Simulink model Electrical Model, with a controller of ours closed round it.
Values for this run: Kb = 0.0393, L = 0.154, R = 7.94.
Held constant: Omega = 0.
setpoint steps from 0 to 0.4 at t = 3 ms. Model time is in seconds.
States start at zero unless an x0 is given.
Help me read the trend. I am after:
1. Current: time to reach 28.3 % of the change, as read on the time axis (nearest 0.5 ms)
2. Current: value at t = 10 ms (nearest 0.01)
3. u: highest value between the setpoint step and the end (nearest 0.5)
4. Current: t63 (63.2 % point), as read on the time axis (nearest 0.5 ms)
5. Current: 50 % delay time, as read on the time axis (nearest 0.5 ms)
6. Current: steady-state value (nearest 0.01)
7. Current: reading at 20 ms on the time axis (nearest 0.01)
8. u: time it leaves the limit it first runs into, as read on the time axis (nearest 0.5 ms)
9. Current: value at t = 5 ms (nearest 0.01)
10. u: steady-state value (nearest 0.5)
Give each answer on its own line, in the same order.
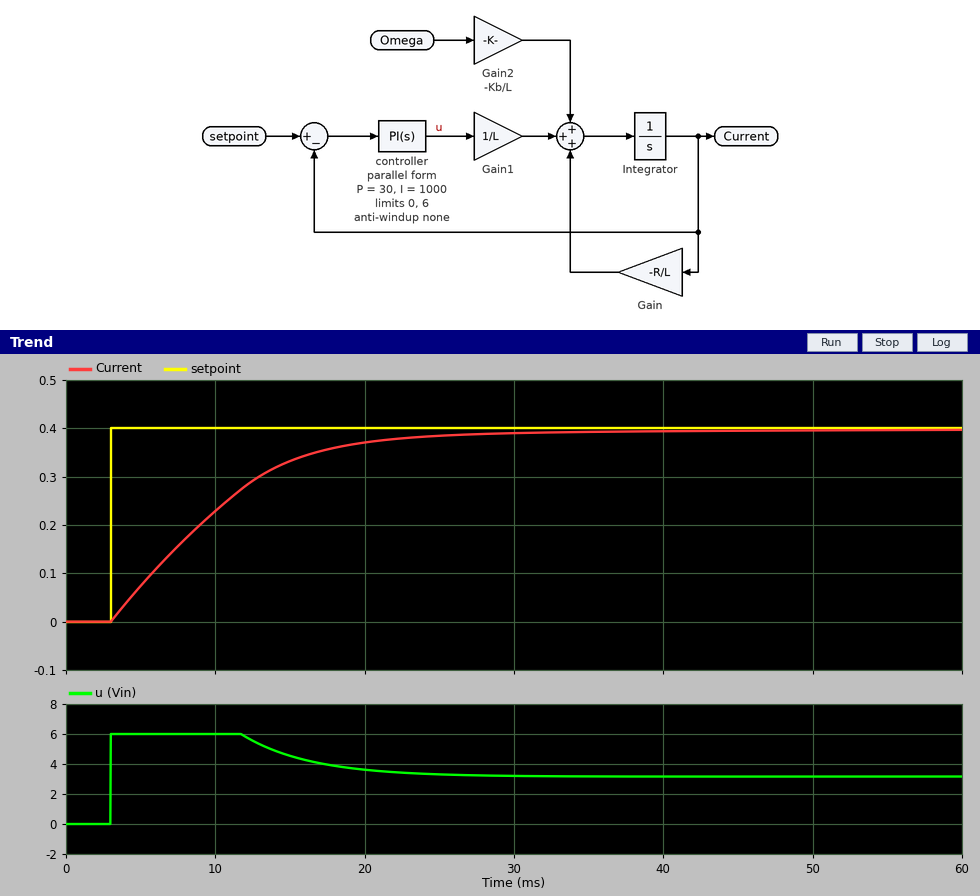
6.0 ms
0.23
6.0
11.0 ms
9.0 ms
0.40
0.37
12.0 ms
0.07
3.0
